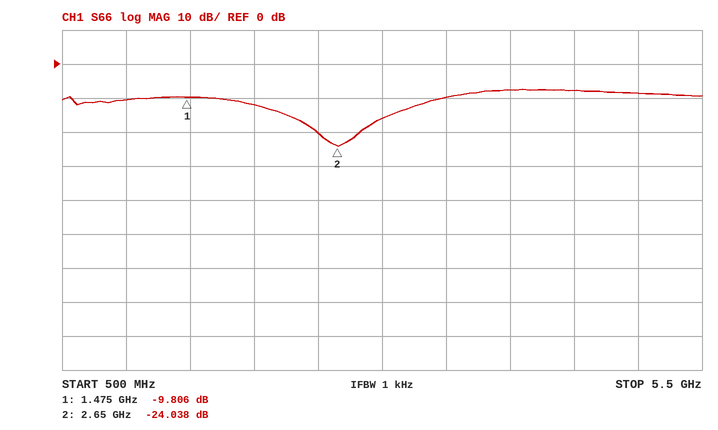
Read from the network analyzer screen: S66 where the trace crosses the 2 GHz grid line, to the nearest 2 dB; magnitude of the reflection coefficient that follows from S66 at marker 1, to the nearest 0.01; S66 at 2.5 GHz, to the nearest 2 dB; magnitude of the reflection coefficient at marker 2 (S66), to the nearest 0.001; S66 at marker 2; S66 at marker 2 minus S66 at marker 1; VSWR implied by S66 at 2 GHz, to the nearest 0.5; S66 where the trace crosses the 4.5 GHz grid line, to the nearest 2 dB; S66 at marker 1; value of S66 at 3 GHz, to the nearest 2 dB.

-12 dB
0.32
-20 dB
0.063
-24.038 dB
-14.232 dB
1.5
-8 dB
-9.806 dB
-16 dB
